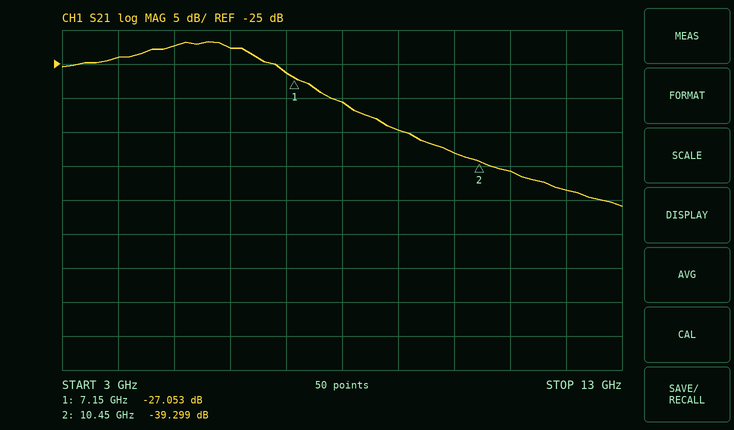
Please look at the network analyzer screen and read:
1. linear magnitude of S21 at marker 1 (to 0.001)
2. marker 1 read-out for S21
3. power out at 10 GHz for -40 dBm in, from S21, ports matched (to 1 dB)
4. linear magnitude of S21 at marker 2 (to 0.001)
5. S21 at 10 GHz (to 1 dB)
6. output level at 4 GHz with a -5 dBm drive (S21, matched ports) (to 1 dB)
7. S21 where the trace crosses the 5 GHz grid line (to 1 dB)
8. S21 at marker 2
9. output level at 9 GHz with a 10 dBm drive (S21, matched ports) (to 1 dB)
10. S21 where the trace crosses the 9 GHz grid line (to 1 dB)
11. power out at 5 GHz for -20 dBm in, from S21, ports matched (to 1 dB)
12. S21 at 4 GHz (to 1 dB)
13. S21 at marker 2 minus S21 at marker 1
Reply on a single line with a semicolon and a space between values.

0.044; -27.053 dB; -78 dBm; 0.011; -38 dB; -29 dBm; -22 dB; -39.299 dB; -25 dBm; -35 dB; -42 dBm; -24 dB; -12.246 dB
